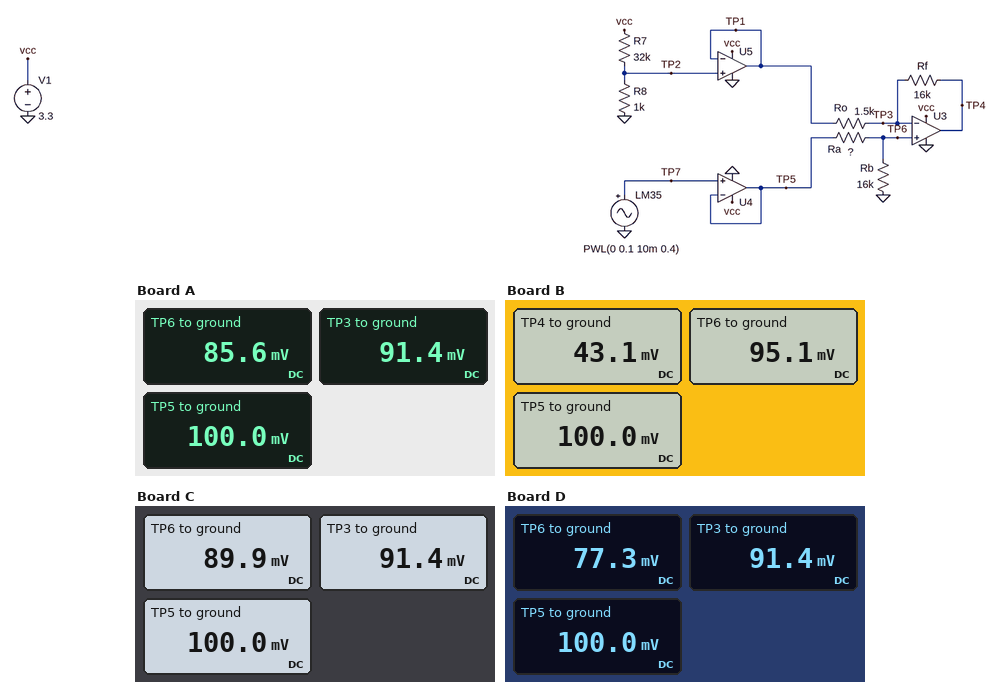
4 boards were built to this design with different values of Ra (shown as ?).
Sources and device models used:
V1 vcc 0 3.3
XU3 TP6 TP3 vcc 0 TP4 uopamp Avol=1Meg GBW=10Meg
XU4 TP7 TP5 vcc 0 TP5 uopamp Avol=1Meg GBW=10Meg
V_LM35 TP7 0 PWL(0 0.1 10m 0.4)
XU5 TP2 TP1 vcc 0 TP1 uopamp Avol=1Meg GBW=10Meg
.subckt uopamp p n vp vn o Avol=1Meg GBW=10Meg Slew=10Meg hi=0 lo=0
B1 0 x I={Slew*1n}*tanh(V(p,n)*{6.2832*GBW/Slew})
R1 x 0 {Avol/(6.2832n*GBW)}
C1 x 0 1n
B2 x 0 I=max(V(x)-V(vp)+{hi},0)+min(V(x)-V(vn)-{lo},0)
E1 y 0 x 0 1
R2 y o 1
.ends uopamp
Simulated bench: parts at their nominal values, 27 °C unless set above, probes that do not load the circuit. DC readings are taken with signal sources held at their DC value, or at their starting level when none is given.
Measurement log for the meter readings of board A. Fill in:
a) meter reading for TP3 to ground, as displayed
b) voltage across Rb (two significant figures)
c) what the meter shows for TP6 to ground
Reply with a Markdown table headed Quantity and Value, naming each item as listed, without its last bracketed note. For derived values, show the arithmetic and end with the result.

| Quantity | Value |
|---|---|
| meter reading for TP3 to ground, as displayed | 91.4 mV |
| voltage across Rb | 85.6 mV = 86 mV |
| what the meter shows for TP6 to ground | 85.6 mV |
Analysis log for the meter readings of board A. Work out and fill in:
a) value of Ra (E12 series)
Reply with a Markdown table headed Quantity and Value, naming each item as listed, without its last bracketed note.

| Quantity | Value |
|---|---|
| value of Ra | 2.7 kΩ |
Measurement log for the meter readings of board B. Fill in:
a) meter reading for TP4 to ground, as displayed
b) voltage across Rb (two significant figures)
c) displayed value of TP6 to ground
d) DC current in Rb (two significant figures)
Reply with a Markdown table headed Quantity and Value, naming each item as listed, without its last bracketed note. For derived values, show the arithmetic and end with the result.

| Quantity | Value |
|---|---|
| meter reading for TP4 to ground, as displayed | 43.1 mV |
| voltage across Rb | 95.1 mV = 95 mV |
| displayed value of TP6 to ground | 95.1 mV |
| DC current in Rb | (95.1 mV) / 16 kΩ = 5.9 µA |
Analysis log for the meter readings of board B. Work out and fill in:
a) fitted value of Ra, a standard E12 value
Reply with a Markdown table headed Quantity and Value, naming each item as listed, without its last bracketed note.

| Quantity | Value |
|---|---|
| fitted value of Ra, a standard E12 value | 820 Ω |
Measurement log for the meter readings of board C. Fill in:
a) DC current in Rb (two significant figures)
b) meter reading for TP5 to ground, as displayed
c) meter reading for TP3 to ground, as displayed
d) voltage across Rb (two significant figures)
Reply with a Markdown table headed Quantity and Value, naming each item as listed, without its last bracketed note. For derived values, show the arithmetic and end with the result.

| Quantity | Value |
|---|---|
| DC current in Rb | (89.9 mV) / 16 kΩ = 5.6 µA |
| meter reading for TP5 to ground, as displayed | 100.0 mV |
| meter reading for TP3 to ground, as displayed | 91.4 mV |
| voltage across Rb | 89.9 mV = 90 mV |
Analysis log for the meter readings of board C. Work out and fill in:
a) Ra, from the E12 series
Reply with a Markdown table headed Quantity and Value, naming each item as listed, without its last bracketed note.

| Quantity | Value |
|---|---|
| Ra, from the E12 series | 1.8 kΩ |
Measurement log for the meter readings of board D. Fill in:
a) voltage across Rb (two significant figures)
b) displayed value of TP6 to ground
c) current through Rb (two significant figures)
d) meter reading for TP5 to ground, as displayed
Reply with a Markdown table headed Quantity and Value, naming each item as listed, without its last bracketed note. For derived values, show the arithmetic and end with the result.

| Quantity | Value |
|---|---|
| voltage across Rb | 77.3 mV = 77 mV |
| displayed value of TP6 to ground | 77.3 mV |
| current through Rb | (77.3 mV) / 16 kΩ = 4.8 µA |
| meter reading for TP5 to ground, as displayed | 100.0 mV |
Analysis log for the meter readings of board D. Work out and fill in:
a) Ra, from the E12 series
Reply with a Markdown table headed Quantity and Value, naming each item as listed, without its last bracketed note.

| Quantity | Value |
|---|---|
| Ra, from the E12 series | 4.7 kΩ |
